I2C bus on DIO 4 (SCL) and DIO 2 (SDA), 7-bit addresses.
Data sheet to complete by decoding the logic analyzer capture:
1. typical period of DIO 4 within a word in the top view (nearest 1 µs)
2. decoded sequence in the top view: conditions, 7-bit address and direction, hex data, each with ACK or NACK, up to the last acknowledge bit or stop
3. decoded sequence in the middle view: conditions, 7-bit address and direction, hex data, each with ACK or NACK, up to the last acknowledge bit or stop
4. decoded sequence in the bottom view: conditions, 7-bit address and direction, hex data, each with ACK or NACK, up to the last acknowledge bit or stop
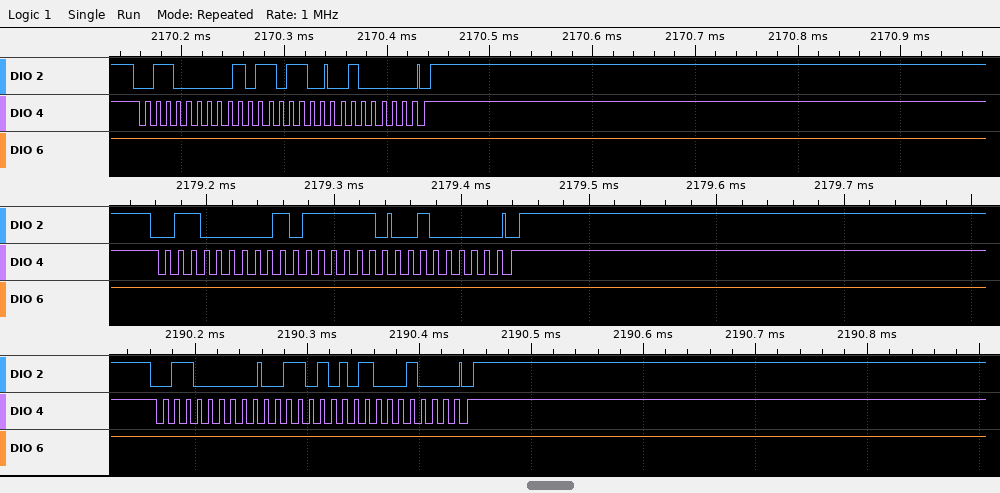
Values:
10 µs
start, address 30 write ACK, B6 ACK, 20 ACK, stop
start, address 30 write ACK, BF ACK, 20 ACK, stop
start, address 30 write ACK, 35 ACK, 88 ACK, stop
